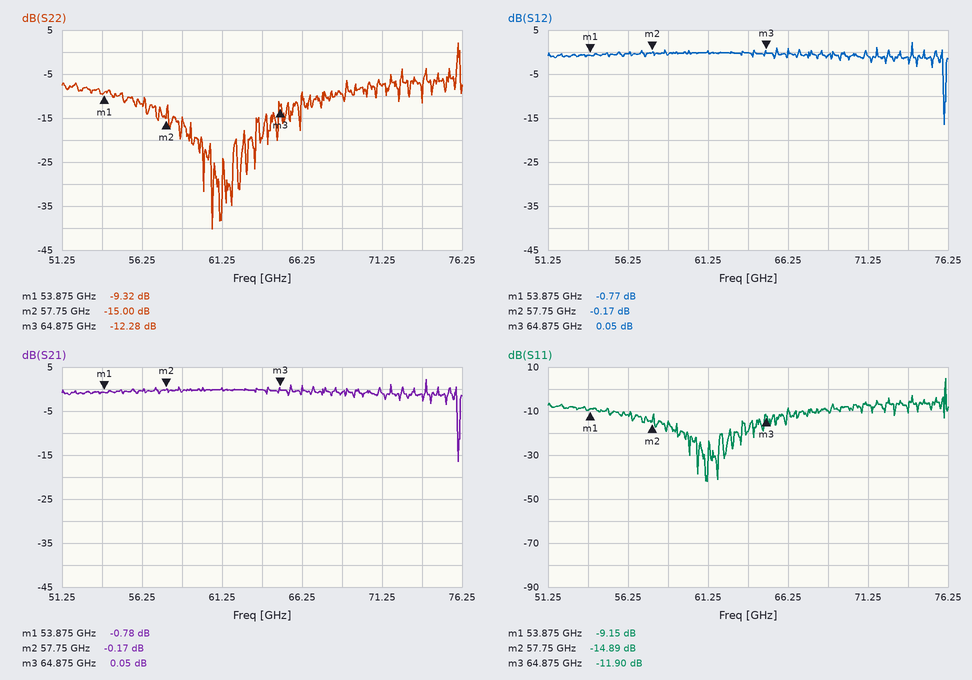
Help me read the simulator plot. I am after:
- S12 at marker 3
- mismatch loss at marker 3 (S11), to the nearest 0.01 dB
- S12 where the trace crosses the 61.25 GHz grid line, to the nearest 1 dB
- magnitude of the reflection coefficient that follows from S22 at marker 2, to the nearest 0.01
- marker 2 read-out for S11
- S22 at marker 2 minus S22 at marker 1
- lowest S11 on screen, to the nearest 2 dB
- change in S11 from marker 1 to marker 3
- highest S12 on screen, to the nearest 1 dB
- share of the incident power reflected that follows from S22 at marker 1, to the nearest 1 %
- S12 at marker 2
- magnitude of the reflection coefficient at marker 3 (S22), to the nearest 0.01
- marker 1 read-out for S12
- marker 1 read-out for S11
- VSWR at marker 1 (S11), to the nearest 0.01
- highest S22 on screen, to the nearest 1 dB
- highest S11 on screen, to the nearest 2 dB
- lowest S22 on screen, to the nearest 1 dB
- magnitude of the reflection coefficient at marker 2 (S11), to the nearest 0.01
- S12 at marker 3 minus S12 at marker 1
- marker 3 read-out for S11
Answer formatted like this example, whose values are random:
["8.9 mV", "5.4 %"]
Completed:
["0.05 dB", "0.29 dB", "0 dB", "0.18", "-14.89 dB", "-5.68 dB", "-42 dB", "-2.75 dB", "2 dB", "12 %", "-0.17 dB", "0.24", "-0.77 dB", "-9.15 dB", "2.07", "2 dB", "4 dB", "-40 dB", "0.18", "0.82 dB", "-11.90 dB"]
